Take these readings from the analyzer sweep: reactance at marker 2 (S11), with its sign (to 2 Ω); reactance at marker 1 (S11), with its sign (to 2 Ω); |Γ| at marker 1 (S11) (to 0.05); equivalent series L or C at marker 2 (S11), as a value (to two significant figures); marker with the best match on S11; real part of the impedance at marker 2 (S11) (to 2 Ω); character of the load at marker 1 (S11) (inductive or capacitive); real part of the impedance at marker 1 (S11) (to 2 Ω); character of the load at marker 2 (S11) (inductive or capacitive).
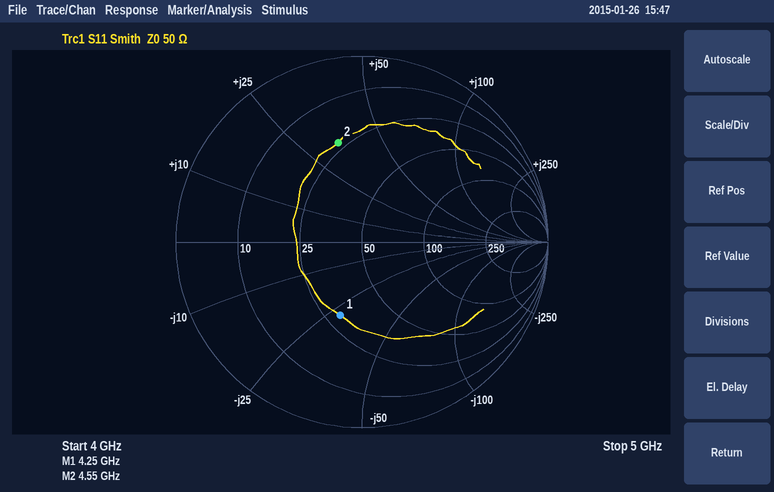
+34 Ω
-28 Ω
0.40
1.2 nH
marker 1
22 Ω
capacitive
30 Ω
inductive
